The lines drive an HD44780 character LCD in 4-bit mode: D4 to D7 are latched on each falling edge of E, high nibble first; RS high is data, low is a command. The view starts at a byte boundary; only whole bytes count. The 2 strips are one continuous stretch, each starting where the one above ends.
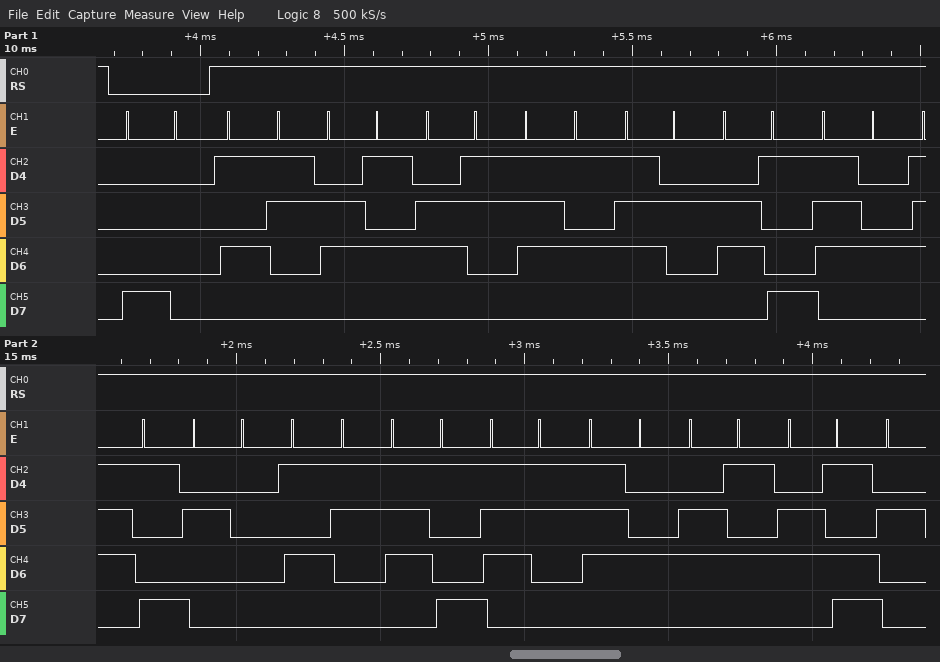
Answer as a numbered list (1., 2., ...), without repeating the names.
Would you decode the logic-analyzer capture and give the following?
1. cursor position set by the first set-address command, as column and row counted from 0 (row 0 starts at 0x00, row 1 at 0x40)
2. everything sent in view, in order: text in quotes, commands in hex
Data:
1. column 0, row 0
2. 0x80 "Security System"
